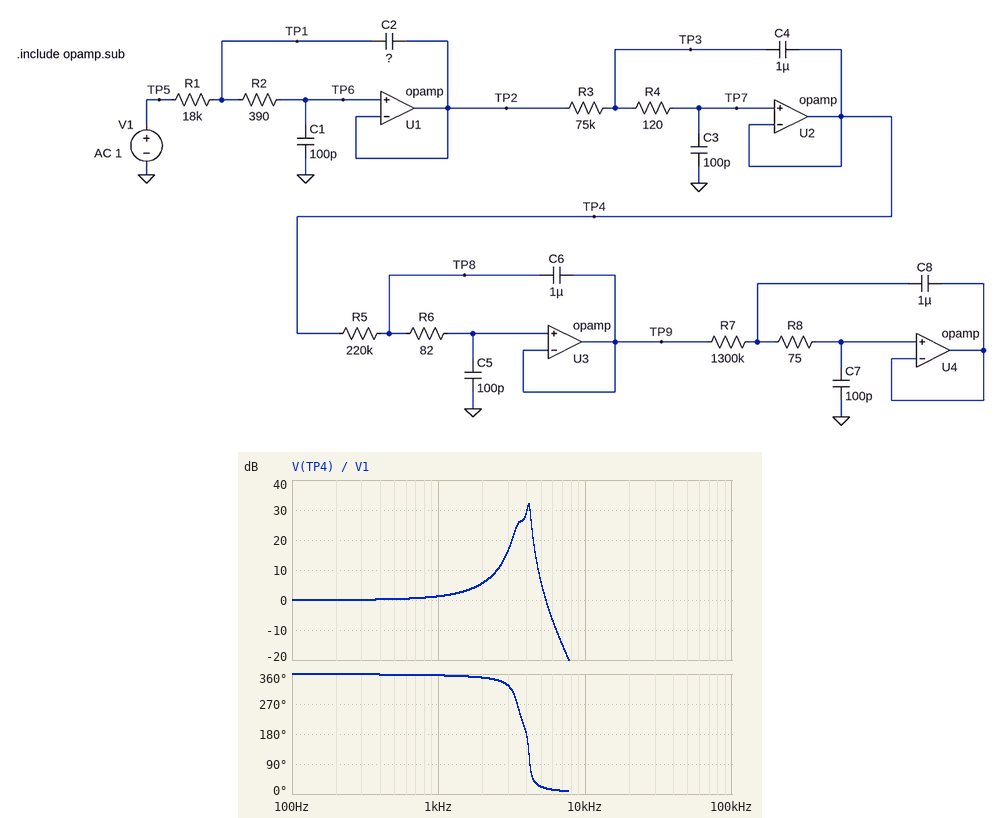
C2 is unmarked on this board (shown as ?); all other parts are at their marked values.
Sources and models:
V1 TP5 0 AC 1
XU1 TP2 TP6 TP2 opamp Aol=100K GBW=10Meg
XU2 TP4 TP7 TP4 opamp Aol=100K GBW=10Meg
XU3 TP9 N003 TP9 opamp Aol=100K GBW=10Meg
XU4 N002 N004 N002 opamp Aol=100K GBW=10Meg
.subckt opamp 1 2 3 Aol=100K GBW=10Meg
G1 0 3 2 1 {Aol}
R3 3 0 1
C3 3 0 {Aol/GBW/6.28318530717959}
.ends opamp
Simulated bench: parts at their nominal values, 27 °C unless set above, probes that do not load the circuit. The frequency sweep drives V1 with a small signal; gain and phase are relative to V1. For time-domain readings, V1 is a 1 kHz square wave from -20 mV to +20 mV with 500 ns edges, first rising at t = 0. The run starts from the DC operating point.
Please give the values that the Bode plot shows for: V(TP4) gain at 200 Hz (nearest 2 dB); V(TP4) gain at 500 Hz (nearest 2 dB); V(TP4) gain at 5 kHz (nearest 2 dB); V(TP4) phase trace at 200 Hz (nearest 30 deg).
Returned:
0 dB
0 dB
6 dB
360 deg
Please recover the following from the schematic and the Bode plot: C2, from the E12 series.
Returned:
1.5 µF
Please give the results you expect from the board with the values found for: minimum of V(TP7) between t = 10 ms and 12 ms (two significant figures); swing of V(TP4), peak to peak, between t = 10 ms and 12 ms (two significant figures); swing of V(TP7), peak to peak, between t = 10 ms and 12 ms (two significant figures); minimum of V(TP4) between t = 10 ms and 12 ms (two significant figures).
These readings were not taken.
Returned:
-82 mV
160 mV
160 mV
-82 mV
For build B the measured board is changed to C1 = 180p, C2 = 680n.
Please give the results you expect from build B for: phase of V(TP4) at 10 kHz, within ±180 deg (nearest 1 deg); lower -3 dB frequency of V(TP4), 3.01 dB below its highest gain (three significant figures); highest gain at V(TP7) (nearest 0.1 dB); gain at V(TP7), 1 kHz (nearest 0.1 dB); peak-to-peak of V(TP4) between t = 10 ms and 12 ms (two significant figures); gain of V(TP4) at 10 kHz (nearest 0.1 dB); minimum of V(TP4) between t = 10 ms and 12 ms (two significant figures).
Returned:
8 deg
3.21 kHz
20.9 dB
1.1 dB
180 mV
-27.3 dB
-89 mV
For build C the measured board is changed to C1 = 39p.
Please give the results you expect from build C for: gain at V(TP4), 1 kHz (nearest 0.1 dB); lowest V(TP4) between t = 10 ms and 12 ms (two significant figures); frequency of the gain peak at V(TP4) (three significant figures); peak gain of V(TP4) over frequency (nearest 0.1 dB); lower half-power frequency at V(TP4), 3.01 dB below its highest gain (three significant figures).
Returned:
1.0 dB
-83 mV
5.48 kHz
25.7 dB
5.38 kHz
